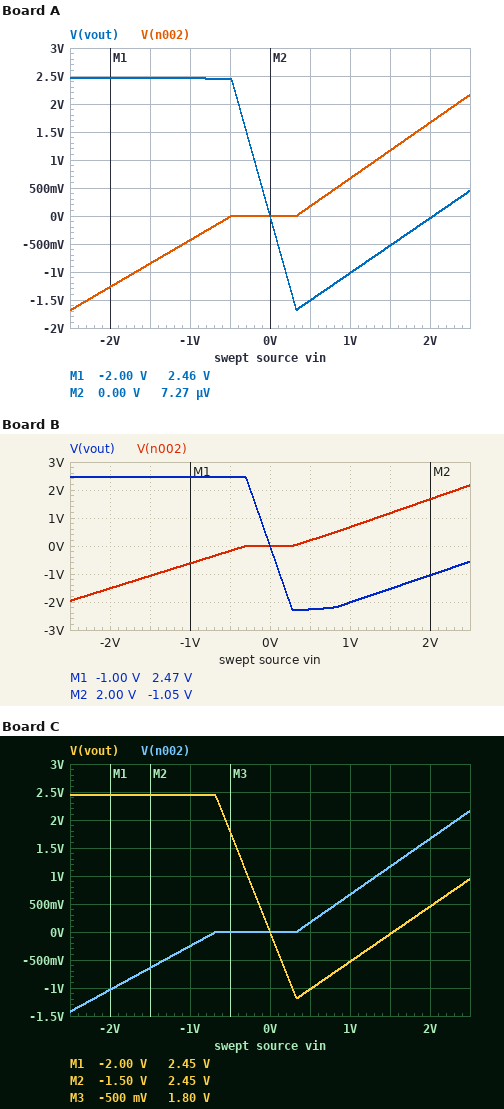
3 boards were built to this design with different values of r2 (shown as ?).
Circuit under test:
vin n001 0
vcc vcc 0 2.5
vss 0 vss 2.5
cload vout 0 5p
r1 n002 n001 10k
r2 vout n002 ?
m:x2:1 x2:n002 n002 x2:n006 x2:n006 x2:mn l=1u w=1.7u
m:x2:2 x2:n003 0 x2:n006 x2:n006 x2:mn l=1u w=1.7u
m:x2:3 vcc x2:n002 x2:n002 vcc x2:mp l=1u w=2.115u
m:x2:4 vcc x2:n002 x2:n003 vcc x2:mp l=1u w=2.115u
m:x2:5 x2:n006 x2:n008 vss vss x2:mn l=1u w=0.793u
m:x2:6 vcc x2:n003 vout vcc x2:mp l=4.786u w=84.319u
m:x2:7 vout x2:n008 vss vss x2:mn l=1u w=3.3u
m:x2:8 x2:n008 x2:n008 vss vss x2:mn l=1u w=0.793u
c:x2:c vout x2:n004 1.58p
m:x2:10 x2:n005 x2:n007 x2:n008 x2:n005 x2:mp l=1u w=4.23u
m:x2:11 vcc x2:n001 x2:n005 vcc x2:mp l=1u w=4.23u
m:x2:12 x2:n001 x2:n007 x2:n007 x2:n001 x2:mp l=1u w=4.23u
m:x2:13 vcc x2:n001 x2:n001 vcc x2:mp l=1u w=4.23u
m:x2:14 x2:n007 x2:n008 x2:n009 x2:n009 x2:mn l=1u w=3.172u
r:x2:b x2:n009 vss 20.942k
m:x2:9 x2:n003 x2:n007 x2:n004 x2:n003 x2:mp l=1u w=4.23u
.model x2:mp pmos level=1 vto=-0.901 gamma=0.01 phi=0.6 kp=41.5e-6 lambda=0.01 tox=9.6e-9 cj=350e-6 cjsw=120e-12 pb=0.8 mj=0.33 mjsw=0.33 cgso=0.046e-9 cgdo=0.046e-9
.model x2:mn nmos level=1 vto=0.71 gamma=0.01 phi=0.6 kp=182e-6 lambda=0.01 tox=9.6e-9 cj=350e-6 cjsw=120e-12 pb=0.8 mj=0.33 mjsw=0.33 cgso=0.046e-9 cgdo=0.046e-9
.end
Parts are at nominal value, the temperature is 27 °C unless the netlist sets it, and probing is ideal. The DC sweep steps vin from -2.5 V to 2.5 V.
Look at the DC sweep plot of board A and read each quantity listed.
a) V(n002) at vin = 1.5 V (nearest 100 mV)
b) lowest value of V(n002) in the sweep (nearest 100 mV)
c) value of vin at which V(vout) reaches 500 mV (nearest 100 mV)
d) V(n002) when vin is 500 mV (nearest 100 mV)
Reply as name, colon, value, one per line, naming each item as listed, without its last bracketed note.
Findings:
V(n002) at vin = 1.5 V: 1.2 V
lowest value of V(n002) in the sweep: -1.7 V
value of vin at which V(vout) reaches 500 mV: -100 mV
V(n002) when vin is 500 mV: 200 mV
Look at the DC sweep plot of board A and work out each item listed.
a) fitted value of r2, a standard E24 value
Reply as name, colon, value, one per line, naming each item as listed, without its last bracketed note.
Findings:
fitted value of r2, a standard E24 value: 51 kΩ
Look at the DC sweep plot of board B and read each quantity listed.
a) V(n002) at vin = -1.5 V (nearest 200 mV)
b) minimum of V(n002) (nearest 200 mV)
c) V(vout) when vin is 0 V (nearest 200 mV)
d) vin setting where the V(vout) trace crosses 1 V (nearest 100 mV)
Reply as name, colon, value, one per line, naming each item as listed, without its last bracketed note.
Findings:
V(n002) at vin = -1.5 V: -1.0 V
minimum of V(n002): -2.0 V
V(vout) when vin is 0 V: 0 V
vin setting where the V(vout) trace crosses 1 V: -100 mV
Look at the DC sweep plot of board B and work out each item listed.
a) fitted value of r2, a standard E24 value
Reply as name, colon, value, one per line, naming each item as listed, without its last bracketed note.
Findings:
fitted value of r2, a standard E24 value: 82 kΩ
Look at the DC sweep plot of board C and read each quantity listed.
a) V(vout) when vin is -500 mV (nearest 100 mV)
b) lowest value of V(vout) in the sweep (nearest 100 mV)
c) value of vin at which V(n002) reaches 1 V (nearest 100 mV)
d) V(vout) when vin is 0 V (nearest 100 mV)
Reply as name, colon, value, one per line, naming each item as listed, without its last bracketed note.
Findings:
V(vout) when vin is -500 mV: 1.8 V
lowest value of V(vout) in the sweep: -1.2 V
value of vin at which V(n002) reaches 1 V: 1.3 V
V(vout) when vin is 0 V: 0 V
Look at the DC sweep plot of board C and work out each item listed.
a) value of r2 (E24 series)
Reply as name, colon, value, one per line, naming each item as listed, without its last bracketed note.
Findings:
value of r2: 36 kΩ
